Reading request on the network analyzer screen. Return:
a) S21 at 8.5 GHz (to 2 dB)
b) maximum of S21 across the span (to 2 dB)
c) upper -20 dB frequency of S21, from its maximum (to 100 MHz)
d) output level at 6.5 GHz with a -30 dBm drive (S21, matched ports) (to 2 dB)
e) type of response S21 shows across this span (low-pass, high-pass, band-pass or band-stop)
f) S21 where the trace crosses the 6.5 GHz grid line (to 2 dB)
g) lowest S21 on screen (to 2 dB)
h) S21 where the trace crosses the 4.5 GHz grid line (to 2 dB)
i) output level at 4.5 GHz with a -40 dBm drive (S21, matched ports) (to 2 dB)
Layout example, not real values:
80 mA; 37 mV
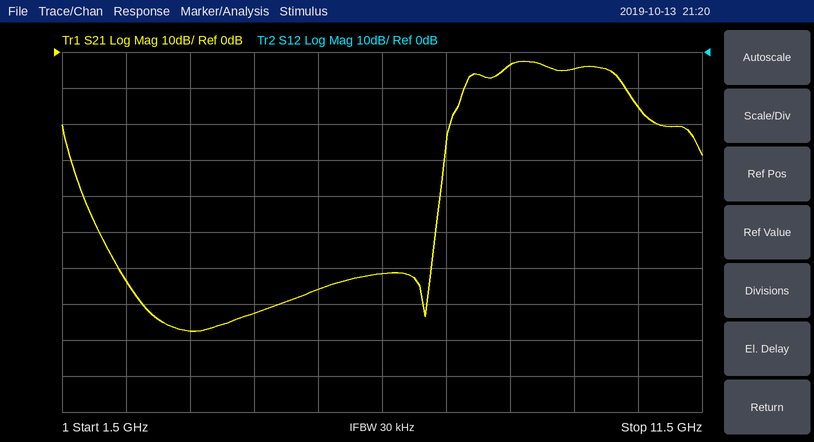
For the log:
-4 dB; -2 dB; 11.3 GHz; -92 dBm; band-pass; -62 dB; -78 dB; -72 dB; -112 dBm
